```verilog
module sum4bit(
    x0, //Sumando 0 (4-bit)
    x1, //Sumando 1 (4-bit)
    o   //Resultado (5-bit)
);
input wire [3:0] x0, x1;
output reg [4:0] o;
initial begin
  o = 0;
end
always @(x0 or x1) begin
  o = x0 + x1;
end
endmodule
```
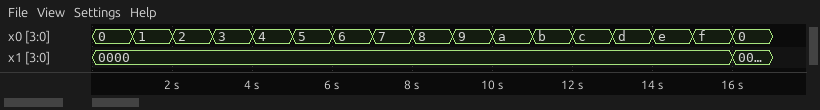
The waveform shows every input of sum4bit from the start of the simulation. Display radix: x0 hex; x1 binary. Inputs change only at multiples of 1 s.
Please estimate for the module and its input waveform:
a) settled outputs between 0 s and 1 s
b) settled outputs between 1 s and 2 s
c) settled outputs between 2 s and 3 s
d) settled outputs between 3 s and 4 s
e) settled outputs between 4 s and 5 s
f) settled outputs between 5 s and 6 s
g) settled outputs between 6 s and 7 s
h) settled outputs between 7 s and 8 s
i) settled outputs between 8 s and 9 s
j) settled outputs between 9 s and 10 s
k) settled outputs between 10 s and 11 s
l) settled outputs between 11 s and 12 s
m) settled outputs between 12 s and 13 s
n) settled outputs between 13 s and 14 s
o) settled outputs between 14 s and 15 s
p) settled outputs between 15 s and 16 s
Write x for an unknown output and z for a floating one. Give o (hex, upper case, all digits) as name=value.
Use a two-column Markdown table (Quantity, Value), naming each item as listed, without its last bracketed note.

| Quantity | Value |
|---|---|
| settled outputs between 0 s and 1 s | o=00 |
| settled outputs between 1 s and 2 s | o=01 |
| settled outputs between 2 s and 3 s | o=02 |
| settled outputs between 3 s and 4 s | o=03 |
| settled outputs between 4 s and 5 s | o=04 |
| settled outputs between 5 s and 6 s | o=05 |
| settled outputs between 6 s and 7 s | o=06 |
| settled outputs between 7 s and 8 s | o=07 |
| settled outputs between 8 s and 9 s | o=08 |
| settled outputs between 9 s and 10 s | o=09 |
| settled outputs between 10 s and 11 s | o=0A |
| settled outputs between 11 s and 12 s | o=0B |
| settled outputs between 12 s and 13 s | o=0C |
| settled outputs between 13 s and 14 s | o=0D |
| settled outputs between 14 s and 15 s | o=0E |
| settled outputs between 15 s and 16 s | o=0F |
